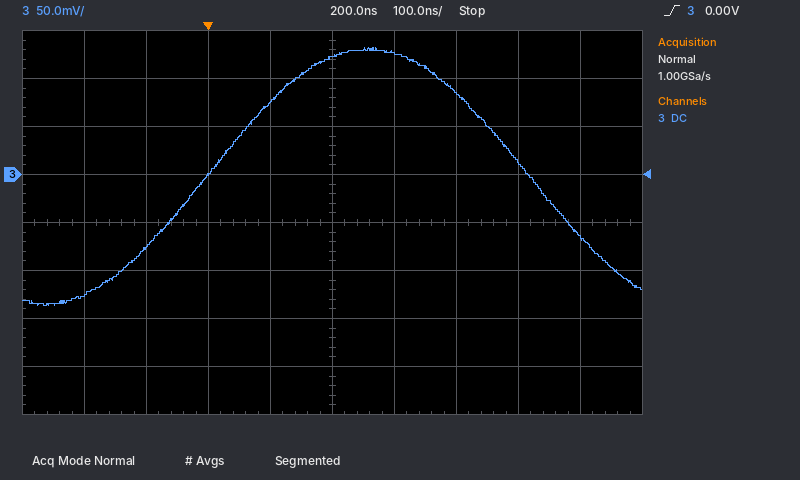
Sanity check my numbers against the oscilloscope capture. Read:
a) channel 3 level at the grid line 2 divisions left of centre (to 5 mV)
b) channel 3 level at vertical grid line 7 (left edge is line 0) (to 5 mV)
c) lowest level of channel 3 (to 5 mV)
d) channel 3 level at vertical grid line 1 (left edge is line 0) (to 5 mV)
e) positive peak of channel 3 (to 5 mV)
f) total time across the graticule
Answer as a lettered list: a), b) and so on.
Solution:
a) 0 mV
b) 85 mV
c) -135 mV
d) -125 mV
e) 130 mV
f) 1 µs
